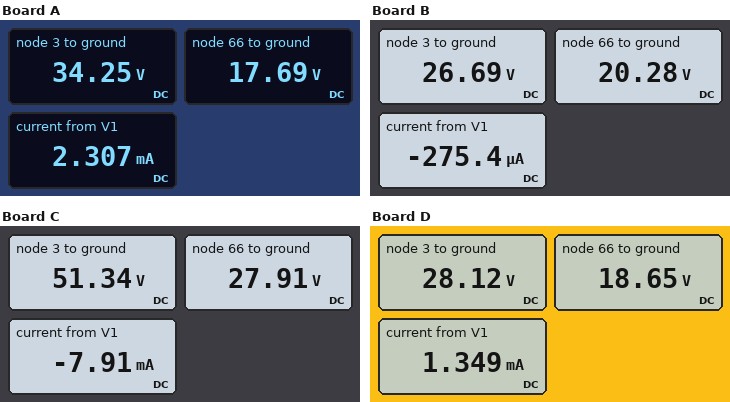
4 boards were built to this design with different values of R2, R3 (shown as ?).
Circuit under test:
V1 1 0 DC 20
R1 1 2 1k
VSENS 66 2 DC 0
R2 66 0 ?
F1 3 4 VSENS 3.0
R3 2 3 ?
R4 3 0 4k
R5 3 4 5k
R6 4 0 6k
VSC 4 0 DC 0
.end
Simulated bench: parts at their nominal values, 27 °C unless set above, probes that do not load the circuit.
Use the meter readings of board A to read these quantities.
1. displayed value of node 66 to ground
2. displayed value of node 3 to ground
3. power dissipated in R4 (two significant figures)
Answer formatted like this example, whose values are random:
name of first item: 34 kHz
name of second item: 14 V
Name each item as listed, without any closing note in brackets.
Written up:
displayed value of node 66 to ground: 17.69 V
displayed value of node 3 to ground: 34.25 V
power dissipated in R4: 290 mW
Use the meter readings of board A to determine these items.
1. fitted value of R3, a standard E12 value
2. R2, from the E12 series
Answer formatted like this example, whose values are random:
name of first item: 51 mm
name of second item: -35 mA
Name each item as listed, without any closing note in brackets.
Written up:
fitted value of R3, a standard E12 value: 3.9 kΩ
R2, from the E12 series: 2.7 kΩ
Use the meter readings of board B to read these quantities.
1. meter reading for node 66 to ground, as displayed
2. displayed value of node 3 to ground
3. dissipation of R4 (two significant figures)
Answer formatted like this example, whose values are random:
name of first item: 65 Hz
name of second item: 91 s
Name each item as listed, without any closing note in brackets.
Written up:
meter reading for node 66 to ground, as displayed: 20.28 V
displayed value of node 3 to ground: 26.69 V
dissipation of R4: 180 mW
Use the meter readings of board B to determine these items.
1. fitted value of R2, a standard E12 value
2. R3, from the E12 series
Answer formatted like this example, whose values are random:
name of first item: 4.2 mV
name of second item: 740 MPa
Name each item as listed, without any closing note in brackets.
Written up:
fitted value of R2, a standard E12 value: 3.3 kΩ
R3, from the E12 series: 1 kΩ
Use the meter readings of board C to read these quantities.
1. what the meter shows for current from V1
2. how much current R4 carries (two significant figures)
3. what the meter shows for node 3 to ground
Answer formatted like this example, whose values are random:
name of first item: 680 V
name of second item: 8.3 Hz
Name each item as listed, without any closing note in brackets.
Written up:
what the meter shows for current from V1: -7.91 mA
how much current R4 carries: 13 mA
what the meter shows for node 3 to ground: 51.34 V
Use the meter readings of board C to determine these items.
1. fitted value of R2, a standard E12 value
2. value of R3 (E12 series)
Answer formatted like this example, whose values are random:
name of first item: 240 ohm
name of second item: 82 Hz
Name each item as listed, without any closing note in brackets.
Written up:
fitted value of R2, a standard E12 value: 1.8 kΩ
value of R3: 1 kΩ
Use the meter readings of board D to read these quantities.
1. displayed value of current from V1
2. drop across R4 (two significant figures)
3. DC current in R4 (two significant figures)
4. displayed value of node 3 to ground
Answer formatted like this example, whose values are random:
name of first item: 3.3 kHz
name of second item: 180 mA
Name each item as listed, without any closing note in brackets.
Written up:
displayed value of current from V1: 1.349 mA
drop across R4: 28 V
DC current in R4: 7.0 mA
displayed value of node 3 to ground: 28.12 V
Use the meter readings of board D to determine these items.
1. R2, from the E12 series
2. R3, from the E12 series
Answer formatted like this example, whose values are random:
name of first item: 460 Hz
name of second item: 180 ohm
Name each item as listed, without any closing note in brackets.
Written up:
R2, from the E12 series: 3.3 kΩ
R3, from the E12 series: 2.2 kΩ
